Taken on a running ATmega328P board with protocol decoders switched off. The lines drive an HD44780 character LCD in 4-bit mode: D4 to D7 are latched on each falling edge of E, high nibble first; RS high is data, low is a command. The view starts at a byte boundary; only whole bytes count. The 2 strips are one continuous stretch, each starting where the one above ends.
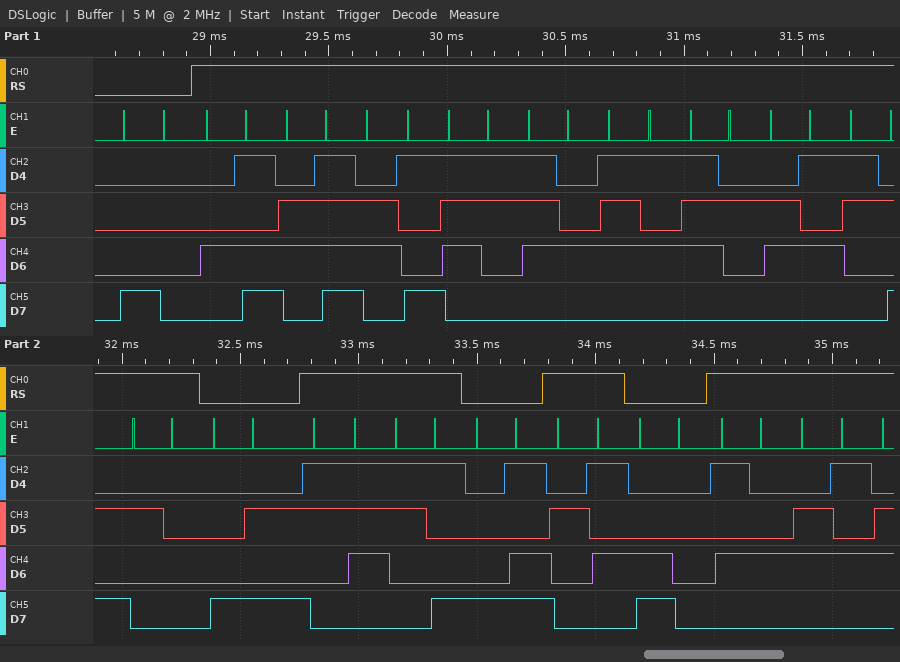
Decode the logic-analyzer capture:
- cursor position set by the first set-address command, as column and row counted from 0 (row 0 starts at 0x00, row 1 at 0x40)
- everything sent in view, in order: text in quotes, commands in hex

column 0, row 0
0x80 "Moisture: " 0x8A "79" 0x8D "%" 0xC0 "Te"
